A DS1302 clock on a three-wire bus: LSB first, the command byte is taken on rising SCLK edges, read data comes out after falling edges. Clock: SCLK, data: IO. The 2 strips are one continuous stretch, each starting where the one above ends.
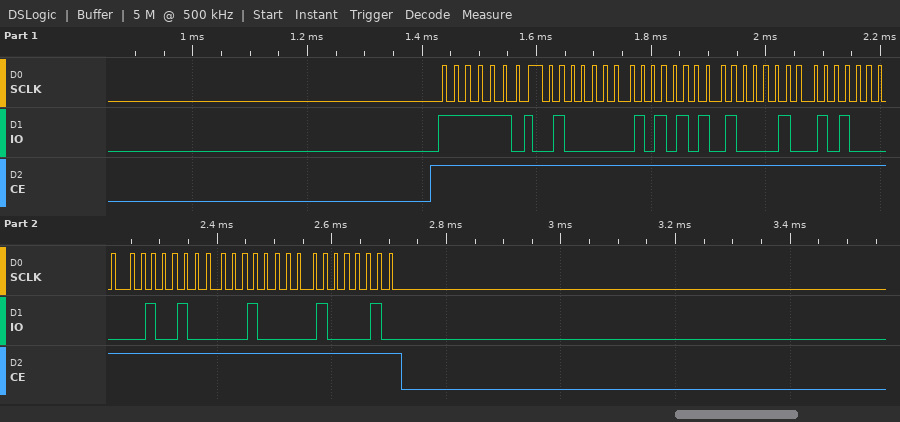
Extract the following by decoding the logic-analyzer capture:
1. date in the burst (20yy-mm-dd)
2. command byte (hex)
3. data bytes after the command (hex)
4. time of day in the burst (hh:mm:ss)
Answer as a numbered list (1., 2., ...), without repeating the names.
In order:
1. 2021-12-05
2. 0xBF
3. 02 55 21 05 12 04 21
4. 21:55:02
